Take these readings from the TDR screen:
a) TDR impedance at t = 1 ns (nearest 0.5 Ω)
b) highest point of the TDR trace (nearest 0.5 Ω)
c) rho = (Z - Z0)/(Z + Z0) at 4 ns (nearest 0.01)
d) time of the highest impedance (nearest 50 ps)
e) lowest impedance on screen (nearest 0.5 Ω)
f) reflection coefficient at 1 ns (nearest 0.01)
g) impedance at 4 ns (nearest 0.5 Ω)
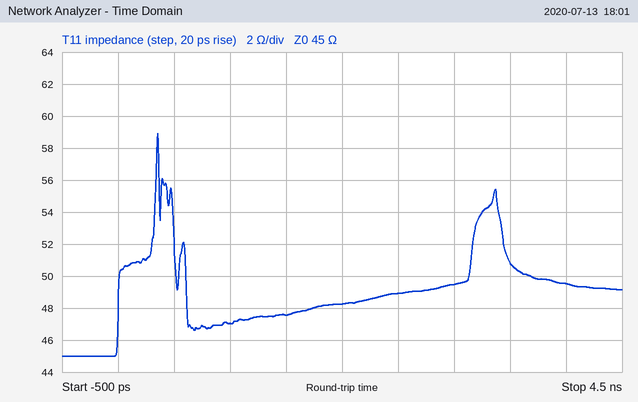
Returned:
47.0 Ω
59.0 Ω
+0.05
350 ps
45.0 Ω
+0.02
49.5 Ω
